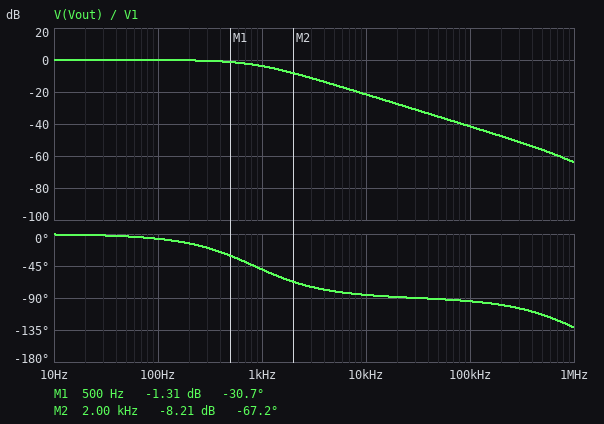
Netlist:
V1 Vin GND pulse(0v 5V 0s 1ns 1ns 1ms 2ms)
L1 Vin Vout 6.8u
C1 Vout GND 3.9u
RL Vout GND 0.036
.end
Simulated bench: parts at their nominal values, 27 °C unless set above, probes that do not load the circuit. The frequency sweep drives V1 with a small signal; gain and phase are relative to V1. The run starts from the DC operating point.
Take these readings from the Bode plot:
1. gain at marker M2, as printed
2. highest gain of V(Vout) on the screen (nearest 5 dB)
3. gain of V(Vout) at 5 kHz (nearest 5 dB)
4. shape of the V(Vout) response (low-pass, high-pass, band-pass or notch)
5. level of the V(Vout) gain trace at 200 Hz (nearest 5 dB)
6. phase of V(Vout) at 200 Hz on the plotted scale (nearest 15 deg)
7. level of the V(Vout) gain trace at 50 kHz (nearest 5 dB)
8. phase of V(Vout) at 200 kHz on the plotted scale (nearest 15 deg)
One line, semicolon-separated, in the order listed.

-8.21 dB; 0 dB; -15 dB; low-pass; 0 dB; -15 deg; -35 dB; -105 deg
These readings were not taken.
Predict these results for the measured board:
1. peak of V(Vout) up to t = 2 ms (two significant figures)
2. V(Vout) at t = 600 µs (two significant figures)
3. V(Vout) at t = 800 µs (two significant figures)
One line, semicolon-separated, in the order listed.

5.0 V; 4.8 V; 4.9 V
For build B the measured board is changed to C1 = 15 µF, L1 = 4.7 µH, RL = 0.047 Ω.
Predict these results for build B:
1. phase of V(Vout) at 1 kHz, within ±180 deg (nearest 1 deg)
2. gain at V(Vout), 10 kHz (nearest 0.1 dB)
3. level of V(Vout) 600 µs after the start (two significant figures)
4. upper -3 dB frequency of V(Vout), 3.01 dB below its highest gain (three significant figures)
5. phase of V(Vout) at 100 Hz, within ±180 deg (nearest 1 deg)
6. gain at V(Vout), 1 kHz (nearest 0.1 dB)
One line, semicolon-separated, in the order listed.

-32 deg; -16.0 dB; 5.0 V; 1.60 kHz; -4 deg; -1.4 dB
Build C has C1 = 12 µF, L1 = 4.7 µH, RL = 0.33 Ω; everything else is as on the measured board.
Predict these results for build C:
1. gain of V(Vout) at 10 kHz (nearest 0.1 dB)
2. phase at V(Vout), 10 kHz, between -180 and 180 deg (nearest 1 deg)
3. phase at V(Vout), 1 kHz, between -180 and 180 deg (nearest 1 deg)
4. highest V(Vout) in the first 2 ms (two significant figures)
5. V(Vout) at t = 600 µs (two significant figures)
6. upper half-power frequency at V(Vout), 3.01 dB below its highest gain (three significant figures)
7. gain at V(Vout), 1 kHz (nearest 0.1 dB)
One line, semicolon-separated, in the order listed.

-1.5 dB; -49 deg; -5 deg; 5.0 V; 5.0 V; 14.7 kHz; 0 dB
